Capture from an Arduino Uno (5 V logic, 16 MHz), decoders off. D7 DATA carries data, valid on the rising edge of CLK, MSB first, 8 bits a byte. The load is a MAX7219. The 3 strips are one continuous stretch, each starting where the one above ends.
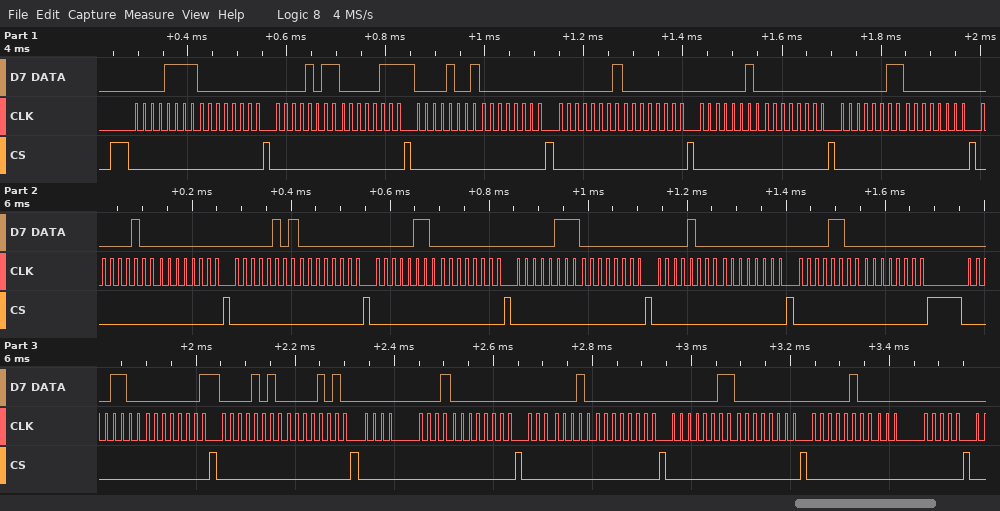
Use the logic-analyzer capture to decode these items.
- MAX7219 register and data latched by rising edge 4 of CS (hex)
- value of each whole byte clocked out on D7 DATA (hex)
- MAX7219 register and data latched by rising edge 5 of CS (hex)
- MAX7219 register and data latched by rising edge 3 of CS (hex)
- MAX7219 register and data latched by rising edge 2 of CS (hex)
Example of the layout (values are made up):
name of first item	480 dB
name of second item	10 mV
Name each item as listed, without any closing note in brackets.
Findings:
MAX7219 register and data latched by rising edge 4 of CS	register 0x9, data 0x00
value of each whole byte clocked out on D7 DATA	0F 00 0B 07 09 00 01 00 02 00 03 00 04 00 05 00 06 00 07 00 08 00 0C 00 0C 01 0A 0A 01 00 02 00 03 00 04 00
MAX7219 register and data latched by rising edge 5 of CS	register 0x1, data 0x00
MAX7219 register and data latched by rising edge 3 of CS	register 0xB, data 0x07
MAX7219 register and data latched by rising edge 2 of CS	register 0xF, data 0x00
